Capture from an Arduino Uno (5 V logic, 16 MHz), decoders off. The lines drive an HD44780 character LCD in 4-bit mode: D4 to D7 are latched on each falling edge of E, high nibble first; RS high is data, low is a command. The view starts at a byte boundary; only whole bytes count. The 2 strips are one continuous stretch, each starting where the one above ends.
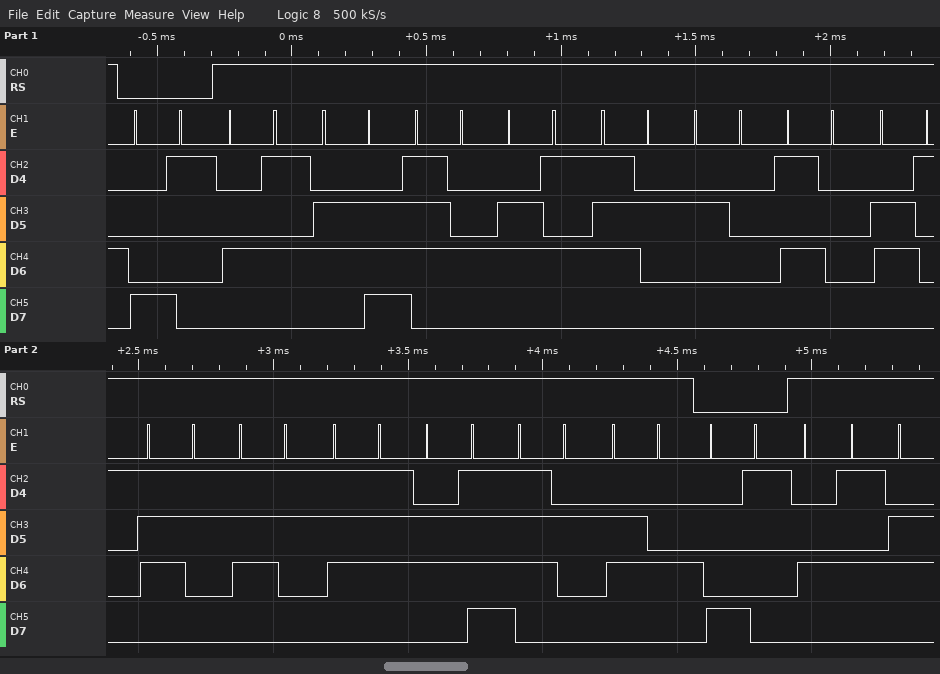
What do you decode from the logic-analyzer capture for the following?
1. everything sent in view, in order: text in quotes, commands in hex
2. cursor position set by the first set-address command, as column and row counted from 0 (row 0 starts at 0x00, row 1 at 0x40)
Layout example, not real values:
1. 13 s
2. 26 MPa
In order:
1. 0x81 "Enter Password" 0x81 "E"
2. column 1, row 0
